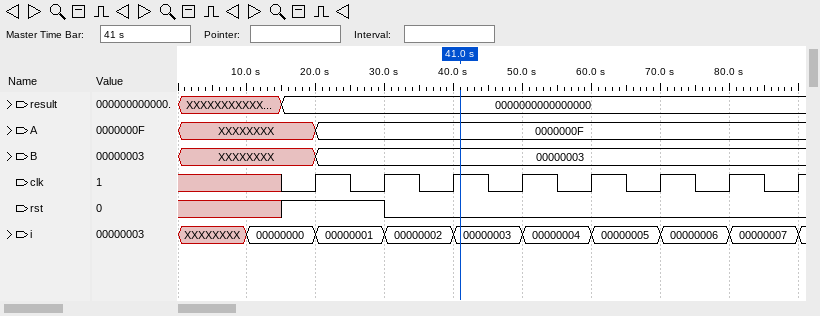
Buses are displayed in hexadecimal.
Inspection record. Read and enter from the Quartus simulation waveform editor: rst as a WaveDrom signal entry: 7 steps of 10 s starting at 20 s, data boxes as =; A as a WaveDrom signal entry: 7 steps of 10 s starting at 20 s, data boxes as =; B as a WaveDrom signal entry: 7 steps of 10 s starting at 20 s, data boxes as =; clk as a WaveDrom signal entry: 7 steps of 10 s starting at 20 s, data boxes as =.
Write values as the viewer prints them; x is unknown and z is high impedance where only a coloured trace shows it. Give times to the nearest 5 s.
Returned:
{name: 'rst', wave: '10.....'}
{name: 'A', wave: '=......', data: '0000000F'}
{name: 'B', wave: '=......', data: '00000003'}
{name: 'clk', wave: 'p......'}
